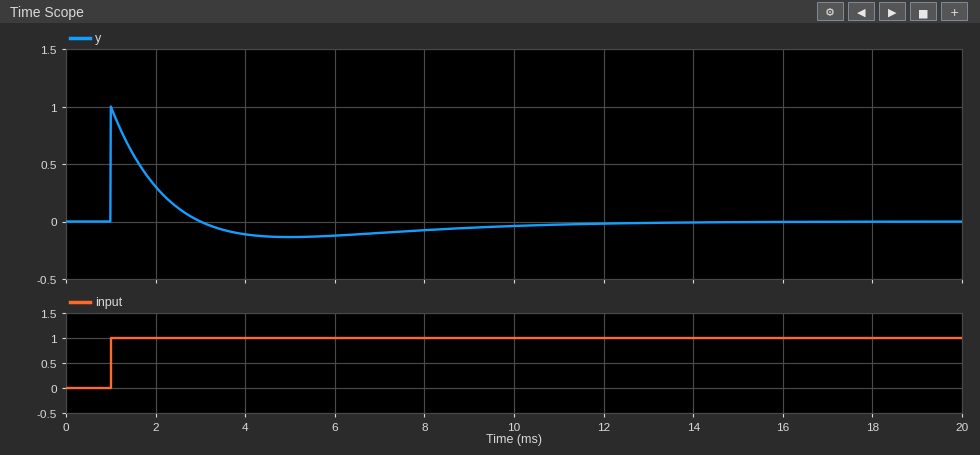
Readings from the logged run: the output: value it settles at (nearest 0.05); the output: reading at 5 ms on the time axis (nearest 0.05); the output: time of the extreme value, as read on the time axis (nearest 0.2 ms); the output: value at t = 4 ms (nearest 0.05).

0.00
-0.15
1.0 ms
-0.10
